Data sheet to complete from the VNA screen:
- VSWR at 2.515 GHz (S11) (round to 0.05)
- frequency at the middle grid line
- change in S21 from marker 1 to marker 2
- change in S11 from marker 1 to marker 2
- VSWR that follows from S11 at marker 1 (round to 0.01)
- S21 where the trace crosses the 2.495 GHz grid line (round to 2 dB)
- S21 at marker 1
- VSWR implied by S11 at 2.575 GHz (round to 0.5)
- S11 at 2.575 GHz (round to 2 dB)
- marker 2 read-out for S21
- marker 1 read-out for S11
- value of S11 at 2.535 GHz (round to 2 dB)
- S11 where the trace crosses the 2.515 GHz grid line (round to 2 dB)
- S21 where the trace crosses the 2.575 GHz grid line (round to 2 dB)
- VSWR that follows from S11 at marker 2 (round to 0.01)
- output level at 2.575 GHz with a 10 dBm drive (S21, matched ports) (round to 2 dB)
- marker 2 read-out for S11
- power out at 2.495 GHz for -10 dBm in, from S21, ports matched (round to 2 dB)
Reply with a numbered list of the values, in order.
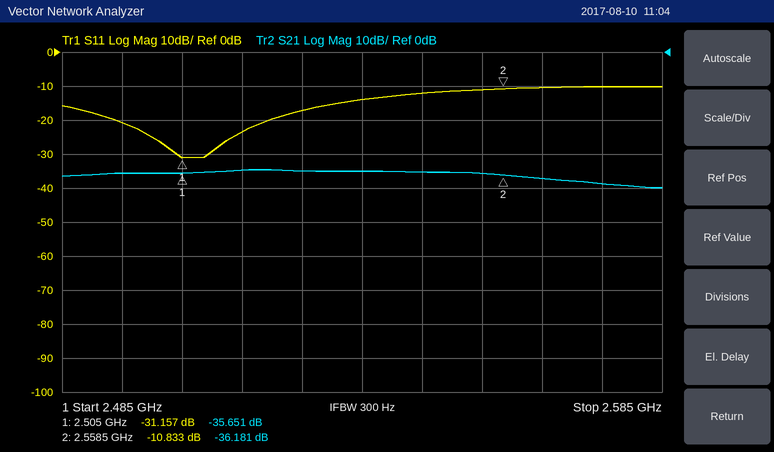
1. 1.15
2. 2.535 GHz
3. -0.530 dB
4. 20.324 dB
5. 1.06
6. -36 dB
7. -35.651 dB
8. 2.0
9. -10 dB
10. -36.181 dB
11. -31.157 dB
12. -14 dB
13. -24 dB
14. -38 dB
15. 1.81
16. -28 dBm
17. -10.833 dB
18. -46 dBm
